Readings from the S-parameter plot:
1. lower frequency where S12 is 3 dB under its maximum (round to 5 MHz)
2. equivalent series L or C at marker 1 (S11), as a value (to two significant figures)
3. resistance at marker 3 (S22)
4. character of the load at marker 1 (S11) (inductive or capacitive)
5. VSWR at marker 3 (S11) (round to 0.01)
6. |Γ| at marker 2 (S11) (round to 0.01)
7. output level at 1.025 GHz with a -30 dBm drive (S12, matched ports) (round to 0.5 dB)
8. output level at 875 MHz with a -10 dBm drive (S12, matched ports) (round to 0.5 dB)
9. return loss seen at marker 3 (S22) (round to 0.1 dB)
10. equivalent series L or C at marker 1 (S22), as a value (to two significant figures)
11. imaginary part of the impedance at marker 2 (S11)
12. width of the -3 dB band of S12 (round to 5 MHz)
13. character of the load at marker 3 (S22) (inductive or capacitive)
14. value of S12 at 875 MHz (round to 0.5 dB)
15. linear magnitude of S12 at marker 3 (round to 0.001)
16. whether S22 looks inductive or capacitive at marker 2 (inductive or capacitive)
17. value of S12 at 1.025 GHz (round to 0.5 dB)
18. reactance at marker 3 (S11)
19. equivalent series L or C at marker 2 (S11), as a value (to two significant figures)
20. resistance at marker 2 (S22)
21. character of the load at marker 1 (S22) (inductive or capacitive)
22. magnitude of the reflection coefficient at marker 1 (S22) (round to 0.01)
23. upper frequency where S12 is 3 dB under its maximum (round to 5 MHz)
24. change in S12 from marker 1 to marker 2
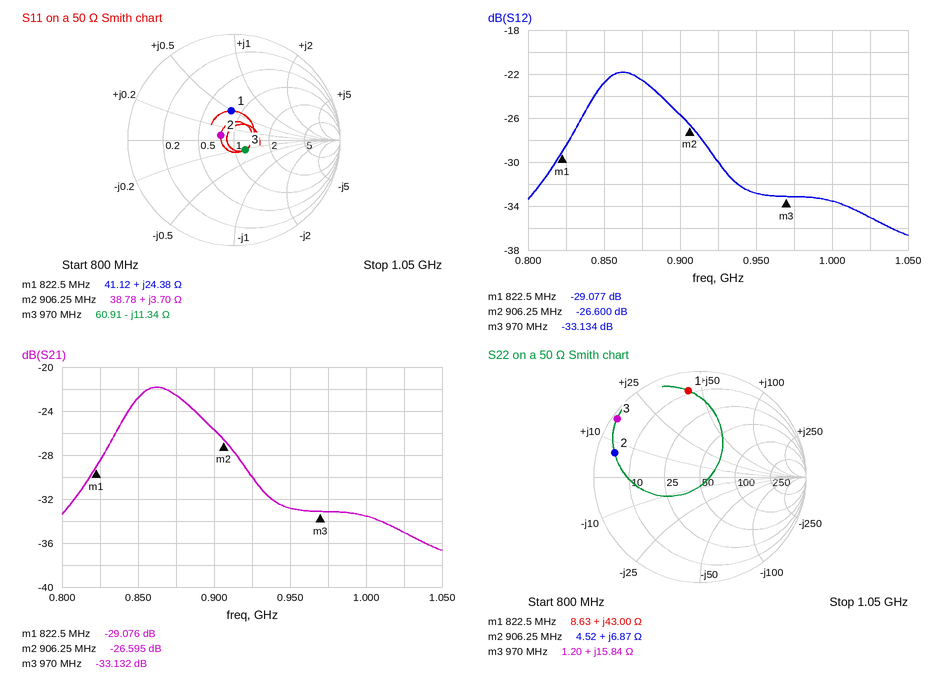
840 MHz
4.7 nH
1.20 Ω
inductive
1.33
0.13
-65.0 dBm
-32.5 dBm
0.4 dB
8.3 nH
+3.70 Ω
55 MHz
inductive
-22.5 dB
0.022
inductive
-35.0 dB
-11.34 Ω
650 pH
4.52 Ω
inductive
0.82
895 MHz
2.477 dB
